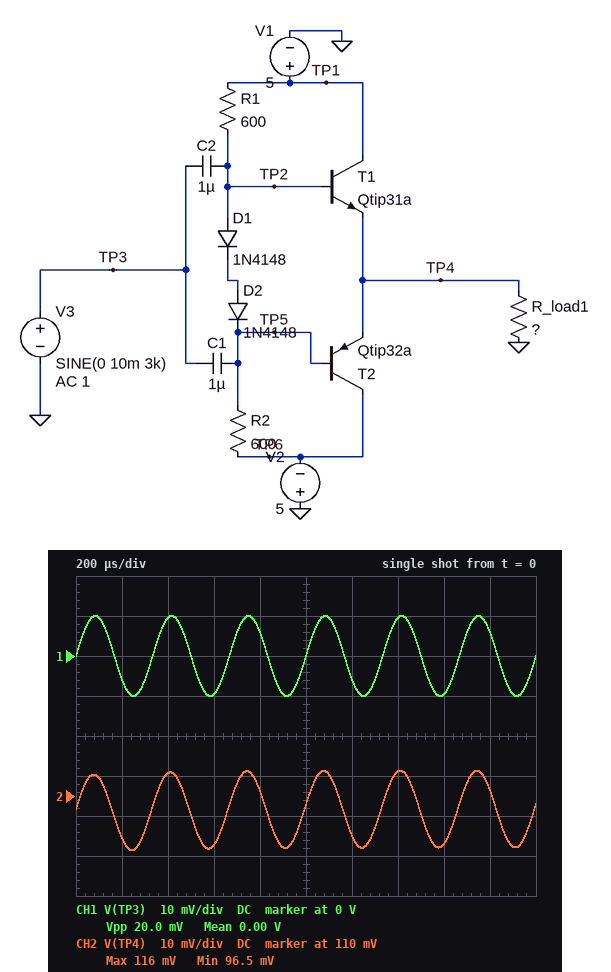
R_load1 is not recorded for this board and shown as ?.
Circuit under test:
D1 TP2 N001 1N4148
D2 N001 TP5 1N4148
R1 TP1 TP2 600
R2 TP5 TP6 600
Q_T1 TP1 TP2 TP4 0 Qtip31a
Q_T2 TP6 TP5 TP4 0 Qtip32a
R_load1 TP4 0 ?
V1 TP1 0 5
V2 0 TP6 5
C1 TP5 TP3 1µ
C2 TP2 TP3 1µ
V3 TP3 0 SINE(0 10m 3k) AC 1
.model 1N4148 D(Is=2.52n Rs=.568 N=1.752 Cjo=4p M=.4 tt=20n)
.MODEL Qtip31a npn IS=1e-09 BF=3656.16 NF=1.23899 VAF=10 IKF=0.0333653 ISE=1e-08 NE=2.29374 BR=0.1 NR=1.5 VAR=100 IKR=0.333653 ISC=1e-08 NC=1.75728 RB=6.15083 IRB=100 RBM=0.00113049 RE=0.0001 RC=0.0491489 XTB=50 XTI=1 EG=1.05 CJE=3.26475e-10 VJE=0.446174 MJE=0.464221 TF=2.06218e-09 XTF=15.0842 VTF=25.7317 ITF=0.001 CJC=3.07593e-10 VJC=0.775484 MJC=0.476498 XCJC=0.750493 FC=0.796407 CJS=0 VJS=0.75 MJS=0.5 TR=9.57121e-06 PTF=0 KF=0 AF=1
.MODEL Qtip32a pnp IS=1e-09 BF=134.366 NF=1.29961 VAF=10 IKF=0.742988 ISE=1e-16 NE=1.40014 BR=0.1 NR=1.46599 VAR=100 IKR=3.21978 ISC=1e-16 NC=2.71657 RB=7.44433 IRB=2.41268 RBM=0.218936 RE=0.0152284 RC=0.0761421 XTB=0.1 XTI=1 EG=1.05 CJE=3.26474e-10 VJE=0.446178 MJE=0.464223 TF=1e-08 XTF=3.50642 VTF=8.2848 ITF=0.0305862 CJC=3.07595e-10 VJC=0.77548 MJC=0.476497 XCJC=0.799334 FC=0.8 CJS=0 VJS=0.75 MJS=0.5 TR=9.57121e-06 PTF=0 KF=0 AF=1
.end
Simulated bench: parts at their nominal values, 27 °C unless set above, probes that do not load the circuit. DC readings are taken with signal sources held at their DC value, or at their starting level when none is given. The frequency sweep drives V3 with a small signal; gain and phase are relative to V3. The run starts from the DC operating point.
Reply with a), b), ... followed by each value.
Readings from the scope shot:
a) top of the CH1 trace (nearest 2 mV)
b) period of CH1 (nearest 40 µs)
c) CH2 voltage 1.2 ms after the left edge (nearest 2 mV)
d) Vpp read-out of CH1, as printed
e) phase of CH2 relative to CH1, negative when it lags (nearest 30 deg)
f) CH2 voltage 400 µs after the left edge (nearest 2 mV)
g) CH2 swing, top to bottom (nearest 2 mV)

a) 10 mV
b) 320 µs
c) 100 mV
d) 20.0 mV
e) 0 deg
f) 116 mV
g) 20 mV
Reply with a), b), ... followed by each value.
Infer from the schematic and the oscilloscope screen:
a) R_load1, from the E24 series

a) 5.1 Ω
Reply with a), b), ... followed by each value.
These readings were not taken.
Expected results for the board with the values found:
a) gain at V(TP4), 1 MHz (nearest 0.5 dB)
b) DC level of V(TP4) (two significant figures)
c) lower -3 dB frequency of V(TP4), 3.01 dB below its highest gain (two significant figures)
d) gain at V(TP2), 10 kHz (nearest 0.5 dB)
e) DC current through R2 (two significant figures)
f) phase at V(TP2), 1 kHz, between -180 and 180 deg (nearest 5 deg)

a) -0.5 dB
b) 110 mV
c) 380 Hz
d) 0 dB
e) 7.4 mA
f) 20 deg
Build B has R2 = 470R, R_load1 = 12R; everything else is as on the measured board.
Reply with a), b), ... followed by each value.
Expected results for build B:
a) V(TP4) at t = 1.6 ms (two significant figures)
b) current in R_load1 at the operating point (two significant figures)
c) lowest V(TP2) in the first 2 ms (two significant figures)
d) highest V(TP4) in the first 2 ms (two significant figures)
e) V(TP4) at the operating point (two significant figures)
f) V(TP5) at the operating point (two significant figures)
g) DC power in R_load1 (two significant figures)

a) -310 mV
b) 25 mA
c) 360 mV
d) -290 mV
e) -300 mV
f) -970 mV
g) 7.6 mW
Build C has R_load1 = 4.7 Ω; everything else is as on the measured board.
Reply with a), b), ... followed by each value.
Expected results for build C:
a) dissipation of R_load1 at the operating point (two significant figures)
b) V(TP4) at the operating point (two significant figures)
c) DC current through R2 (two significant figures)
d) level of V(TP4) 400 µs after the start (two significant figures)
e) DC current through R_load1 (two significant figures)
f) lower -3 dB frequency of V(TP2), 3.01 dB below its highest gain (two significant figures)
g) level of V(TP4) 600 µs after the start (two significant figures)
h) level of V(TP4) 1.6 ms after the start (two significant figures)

a) 2.3 mW
b) 100 mV
c) 7.4 mA
d) 110 mV
e) 22 mA
f) 390 Hz
g) 95 mV
h) 96 mV
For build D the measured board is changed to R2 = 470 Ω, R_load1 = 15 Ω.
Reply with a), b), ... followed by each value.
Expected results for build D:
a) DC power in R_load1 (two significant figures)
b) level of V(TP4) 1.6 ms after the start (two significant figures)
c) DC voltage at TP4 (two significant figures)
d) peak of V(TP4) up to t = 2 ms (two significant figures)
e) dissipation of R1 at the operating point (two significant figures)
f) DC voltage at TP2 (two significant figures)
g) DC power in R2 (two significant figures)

a) 6.4 mW
b) -320 mV
c) -310 mV
d) -300 mV
e) 36 mW
f) 370 mV
g) 34 mW
